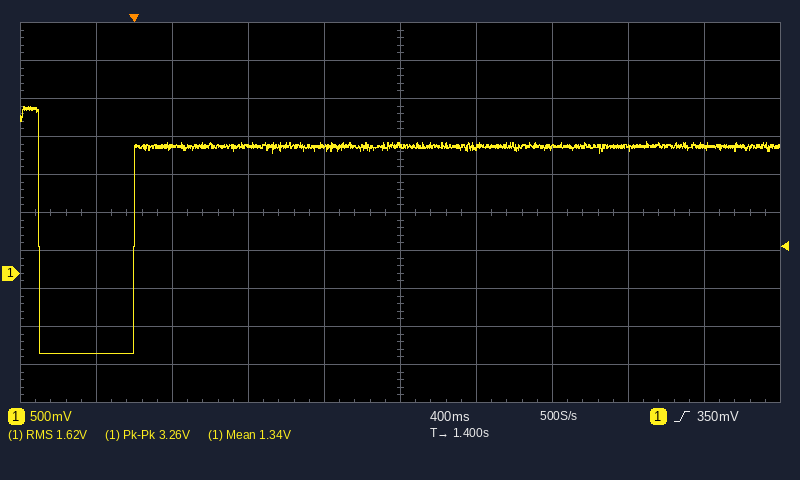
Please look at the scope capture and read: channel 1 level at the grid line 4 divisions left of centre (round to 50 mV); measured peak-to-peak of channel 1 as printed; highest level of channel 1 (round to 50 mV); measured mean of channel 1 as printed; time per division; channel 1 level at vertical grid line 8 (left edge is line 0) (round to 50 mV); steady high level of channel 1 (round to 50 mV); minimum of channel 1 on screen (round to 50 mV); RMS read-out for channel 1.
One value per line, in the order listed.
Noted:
-1.05 V
3.26 V
2.20 V
1.34 V
400 ms
1.65 V
1.65 V
-1.05 V
1.62 V
